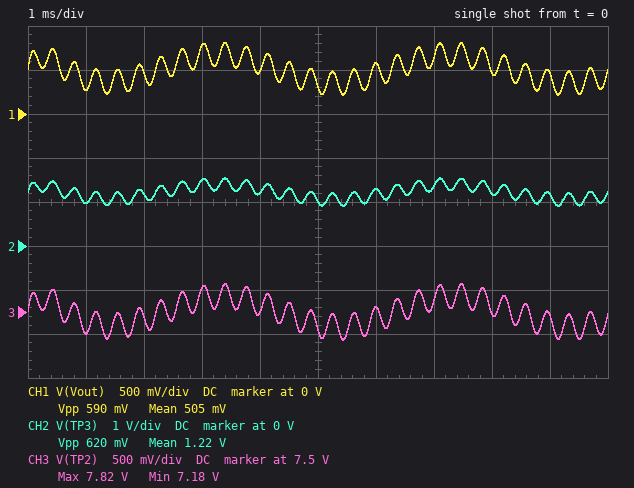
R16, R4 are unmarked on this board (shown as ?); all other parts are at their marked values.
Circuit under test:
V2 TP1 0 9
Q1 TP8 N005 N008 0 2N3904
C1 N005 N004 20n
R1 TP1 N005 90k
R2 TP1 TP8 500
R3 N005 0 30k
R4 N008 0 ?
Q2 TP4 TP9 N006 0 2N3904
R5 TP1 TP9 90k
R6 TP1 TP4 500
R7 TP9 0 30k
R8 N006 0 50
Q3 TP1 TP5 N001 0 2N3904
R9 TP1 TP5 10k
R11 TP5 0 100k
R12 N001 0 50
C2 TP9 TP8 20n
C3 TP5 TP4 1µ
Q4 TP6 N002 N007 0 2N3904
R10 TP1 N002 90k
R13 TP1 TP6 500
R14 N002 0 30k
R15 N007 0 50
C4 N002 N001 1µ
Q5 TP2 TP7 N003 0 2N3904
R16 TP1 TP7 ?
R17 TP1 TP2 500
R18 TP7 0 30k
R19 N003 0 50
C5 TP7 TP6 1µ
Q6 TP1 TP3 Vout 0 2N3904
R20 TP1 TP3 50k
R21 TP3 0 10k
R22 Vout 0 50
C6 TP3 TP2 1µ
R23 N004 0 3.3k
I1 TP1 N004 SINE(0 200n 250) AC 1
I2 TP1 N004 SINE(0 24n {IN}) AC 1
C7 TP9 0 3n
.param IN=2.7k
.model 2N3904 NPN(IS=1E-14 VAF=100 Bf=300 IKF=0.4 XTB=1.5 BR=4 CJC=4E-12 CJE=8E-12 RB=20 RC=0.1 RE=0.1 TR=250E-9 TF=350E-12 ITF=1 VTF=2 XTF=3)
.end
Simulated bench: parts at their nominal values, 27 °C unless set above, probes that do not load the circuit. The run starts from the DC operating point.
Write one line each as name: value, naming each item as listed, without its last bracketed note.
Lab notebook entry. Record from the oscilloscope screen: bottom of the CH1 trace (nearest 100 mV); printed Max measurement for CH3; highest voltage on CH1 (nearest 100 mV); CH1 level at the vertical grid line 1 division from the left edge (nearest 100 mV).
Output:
bottom of the CH1 trace: 200 mV
printed Max measurement for CH3: 7.82 V
highest voltage on CH1: 800 mV
CH1 level at the vertical grid line 1 division from the left edge: 300 mV
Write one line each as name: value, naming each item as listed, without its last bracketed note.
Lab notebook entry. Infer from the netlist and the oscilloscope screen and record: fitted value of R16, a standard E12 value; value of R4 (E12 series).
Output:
fitted value of R16, a standard E12 value: 220 kΩ
value of R4: 100 Ω
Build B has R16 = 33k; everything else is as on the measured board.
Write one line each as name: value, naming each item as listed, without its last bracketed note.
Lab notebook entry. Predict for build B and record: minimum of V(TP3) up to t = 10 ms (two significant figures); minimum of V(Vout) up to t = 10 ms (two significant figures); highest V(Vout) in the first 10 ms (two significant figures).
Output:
minimum of V(TP3) up to t = 10 ms: 1.2 V
minimum of V(Vout) up to t = 10 ms: 510 mV
highest V(Vout) in the first 10 ms: 530 mV
